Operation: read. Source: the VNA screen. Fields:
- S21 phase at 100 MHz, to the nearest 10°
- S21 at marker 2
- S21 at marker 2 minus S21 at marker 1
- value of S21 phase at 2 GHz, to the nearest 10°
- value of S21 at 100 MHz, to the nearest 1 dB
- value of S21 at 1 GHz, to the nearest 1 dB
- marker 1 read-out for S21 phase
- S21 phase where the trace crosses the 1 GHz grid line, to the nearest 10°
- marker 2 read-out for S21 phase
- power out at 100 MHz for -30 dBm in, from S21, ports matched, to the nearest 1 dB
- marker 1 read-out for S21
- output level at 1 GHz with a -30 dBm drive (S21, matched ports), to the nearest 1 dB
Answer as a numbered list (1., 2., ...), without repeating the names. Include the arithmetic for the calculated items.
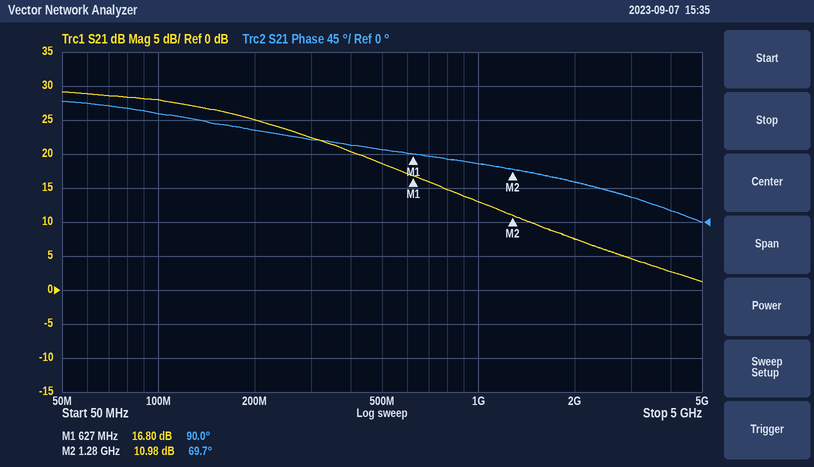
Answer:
1. 140°
2. 10.98 dB
3. 10.98 − (16.8) = -5.82 dB
4. 50°
5. 28 dB
6. 13 dB
7. 90.0°
8. 80°
9. 69.7°
10. -30 dBm + (28 dB) = -2 dBm
11. 16.80 dB
12. -30 dBm + (13 dB) = -17 dBm
